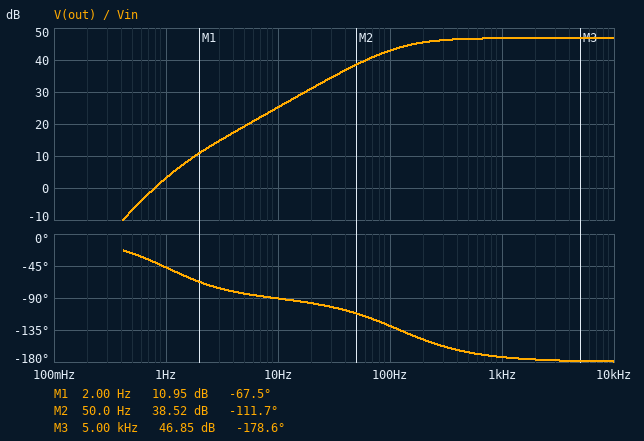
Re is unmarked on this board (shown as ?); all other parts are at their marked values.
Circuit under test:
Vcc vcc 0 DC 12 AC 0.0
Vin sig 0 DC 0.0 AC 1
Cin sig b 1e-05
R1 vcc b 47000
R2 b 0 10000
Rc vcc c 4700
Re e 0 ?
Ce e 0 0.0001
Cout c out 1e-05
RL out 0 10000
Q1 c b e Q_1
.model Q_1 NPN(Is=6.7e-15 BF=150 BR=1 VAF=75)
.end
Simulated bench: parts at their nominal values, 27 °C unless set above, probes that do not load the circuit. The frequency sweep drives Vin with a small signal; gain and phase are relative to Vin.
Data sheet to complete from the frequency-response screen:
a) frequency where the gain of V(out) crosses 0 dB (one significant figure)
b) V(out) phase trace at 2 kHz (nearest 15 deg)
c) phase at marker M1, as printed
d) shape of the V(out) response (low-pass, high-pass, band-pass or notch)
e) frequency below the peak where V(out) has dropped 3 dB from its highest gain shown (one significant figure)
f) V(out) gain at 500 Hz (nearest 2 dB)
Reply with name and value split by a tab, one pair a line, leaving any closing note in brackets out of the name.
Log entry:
frequency where the gain of V(out) crosses 0 dB	800 mHz
V(out) phase trace at 2 kHz	-180 deg
phase at marker M1, as printed	-67.5 deg
shape of the V(out) response	high-pass
frequency below the peak where V(out) has dropped 3 dB from its highest gain shown	100 Hz
V(out) gain at 500 Hz	46 dB
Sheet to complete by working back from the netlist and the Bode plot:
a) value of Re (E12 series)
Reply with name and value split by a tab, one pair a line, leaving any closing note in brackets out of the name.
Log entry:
value of Re	680 Ω
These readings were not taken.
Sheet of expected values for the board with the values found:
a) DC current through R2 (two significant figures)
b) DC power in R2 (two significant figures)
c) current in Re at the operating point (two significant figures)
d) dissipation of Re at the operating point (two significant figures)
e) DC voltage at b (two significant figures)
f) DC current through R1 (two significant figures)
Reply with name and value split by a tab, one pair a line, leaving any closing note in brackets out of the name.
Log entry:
DC current through R2	200 µA
DC power in R2	400 µW
current in Re at the operating point	1.9 mA
dissipation of Re at the operating point	2.6 mW
DC voltage at b	2.0 V
DC current through R1	210 µA
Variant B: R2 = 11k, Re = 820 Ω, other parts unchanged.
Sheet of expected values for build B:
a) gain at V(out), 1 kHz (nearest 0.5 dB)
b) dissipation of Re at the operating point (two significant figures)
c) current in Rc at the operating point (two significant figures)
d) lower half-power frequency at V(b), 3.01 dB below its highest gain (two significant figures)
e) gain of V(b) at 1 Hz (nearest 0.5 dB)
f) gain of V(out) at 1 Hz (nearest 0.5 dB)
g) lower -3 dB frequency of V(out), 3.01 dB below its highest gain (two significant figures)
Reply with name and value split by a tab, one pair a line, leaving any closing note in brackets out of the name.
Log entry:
gain at V(out), 1 kHz	46.5 dB
dissipation of Re at the operating point	2.7 mW
current in Rc at the operating point	1.8 mA
lower half-power frequency at V(b), 3.01 dB below its highest gain	2.1 Hz
gain of V(b) at 1 Hz	-7.0 dB
gain of V(out) at 1 Hz	2.5 dB
lower -3 dB frequency of V(out), 3.01 dB below its highest gain	110 Hz
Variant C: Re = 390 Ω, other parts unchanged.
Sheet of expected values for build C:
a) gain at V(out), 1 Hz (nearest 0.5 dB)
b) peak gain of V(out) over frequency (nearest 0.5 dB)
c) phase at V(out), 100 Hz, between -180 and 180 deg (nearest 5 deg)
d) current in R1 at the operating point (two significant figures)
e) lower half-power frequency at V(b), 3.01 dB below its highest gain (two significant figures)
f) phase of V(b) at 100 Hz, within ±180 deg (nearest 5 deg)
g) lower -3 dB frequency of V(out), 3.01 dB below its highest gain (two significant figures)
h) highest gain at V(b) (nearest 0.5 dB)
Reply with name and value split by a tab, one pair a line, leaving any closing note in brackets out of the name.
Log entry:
gain at V(out), 1 Hz	-43.5 dB
peak gain of V(out) over frequency	28.0 dB
phase at V(out), 100 Hz, between -180 and 180 deg	-95 deg
current in R1 at the operating point	220 µA
lower half-power frequency at V(b), 3.01 dB below its highest gain	760 Hz
phase of V(b) at 100 Hz, within ±180 deg	45 deg
lower -3 dB frequency of V(out), 3.01 dB below its highest gain	770 Hz
highest gain at V(b)	0 dB
